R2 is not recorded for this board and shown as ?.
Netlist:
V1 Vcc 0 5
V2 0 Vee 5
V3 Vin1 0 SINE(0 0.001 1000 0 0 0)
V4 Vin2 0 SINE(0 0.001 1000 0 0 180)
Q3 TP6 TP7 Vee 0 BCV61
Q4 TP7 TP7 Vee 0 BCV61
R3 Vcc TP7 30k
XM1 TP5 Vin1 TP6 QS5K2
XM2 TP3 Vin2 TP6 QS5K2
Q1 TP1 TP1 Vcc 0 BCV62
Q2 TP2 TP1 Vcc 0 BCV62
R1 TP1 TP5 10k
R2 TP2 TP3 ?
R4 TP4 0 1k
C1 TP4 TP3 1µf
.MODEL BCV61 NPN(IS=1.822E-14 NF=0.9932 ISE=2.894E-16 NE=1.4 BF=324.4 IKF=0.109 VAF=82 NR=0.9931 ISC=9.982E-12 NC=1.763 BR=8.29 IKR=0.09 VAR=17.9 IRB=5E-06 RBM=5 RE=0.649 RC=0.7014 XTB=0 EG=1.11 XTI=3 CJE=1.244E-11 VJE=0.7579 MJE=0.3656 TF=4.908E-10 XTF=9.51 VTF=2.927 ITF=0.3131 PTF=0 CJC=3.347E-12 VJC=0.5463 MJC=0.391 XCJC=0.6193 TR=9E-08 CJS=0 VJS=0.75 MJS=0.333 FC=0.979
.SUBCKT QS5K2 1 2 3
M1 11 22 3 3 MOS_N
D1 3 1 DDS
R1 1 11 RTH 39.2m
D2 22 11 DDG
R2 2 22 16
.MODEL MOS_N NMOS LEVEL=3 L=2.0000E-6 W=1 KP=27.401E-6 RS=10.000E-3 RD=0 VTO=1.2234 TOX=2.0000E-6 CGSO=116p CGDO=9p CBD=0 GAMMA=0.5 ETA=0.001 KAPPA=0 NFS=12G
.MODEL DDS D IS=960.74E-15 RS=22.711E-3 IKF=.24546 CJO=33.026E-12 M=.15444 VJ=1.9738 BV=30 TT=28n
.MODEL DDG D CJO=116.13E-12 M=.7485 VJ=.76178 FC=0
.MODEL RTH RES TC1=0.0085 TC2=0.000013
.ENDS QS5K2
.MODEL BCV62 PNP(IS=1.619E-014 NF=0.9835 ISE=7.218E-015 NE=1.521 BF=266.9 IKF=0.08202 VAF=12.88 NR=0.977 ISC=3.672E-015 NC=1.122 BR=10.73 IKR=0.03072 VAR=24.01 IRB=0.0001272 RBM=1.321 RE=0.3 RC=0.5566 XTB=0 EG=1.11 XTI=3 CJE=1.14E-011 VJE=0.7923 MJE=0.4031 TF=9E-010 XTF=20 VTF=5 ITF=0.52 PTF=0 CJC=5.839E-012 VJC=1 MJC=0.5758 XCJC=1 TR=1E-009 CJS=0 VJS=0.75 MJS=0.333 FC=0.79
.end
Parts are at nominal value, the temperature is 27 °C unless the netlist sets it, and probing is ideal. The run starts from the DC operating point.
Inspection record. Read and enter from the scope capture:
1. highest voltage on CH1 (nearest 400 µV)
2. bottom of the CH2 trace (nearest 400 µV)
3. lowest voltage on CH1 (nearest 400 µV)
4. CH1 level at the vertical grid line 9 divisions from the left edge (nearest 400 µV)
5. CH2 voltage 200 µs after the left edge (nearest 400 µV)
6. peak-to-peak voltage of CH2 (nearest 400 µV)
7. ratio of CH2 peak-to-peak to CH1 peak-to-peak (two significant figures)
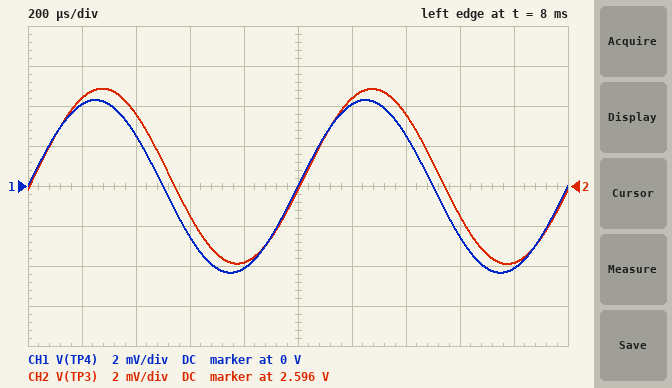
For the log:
4.4 mV
2.5920 V
-4.4 mV
-4.0 mV
2.6004 V
8.8 mV
1.0
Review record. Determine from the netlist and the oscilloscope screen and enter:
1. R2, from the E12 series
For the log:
12 kΩ
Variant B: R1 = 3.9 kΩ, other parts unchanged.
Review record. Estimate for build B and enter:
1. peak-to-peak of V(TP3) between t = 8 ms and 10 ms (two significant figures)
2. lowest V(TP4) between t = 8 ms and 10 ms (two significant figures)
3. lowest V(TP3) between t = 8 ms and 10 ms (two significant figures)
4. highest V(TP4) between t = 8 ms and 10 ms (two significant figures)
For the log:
6.4 mV
-3.2 mV
3.0 V
3.0 mV
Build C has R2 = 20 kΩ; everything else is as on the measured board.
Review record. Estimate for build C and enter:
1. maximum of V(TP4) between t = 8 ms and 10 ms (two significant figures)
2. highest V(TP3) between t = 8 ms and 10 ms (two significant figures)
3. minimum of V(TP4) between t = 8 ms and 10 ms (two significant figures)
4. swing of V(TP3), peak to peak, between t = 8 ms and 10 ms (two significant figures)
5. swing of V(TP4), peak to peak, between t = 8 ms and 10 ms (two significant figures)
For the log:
2.6 mV
1.8 V
-2.7 mV
5.4 mV
5.3 mV
